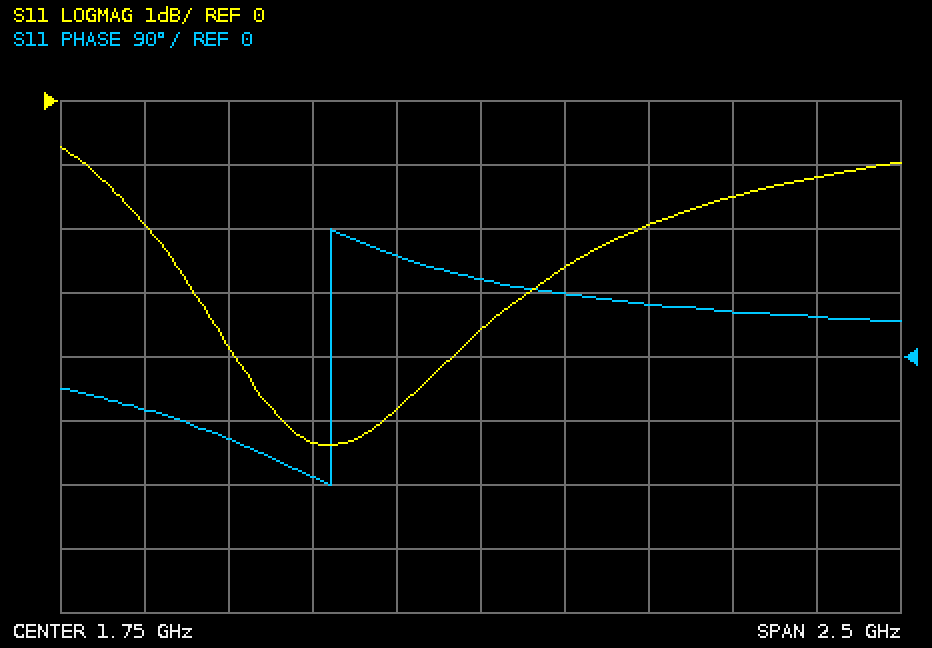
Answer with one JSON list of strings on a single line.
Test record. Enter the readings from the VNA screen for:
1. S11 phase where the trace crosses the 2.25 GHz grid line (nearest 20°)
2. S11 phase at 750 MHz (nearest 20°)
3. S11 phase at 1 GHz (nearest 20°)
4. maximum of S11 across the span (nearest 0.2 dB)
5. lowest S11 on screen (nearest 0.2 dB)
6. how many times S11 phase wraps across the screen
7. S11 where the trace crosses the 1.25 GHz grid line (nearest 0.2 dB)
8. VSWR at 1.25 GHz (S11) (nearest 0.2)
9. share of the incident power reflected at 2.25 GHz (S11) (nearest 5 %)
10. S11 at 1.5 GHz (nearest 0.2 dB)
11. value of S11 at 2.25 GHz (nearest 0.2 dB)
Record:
["80°", "-80°", "-120°", "-0.8 dB", "-5.4 dB", "1", "-5.4 dB", "3.4", "65 %", "-4.8 dB", "-2.0 dB"]
